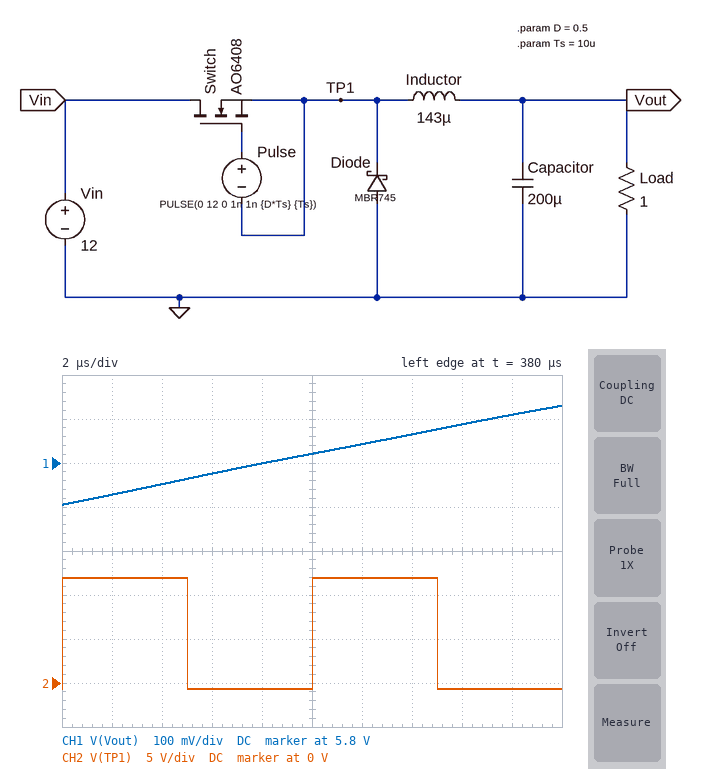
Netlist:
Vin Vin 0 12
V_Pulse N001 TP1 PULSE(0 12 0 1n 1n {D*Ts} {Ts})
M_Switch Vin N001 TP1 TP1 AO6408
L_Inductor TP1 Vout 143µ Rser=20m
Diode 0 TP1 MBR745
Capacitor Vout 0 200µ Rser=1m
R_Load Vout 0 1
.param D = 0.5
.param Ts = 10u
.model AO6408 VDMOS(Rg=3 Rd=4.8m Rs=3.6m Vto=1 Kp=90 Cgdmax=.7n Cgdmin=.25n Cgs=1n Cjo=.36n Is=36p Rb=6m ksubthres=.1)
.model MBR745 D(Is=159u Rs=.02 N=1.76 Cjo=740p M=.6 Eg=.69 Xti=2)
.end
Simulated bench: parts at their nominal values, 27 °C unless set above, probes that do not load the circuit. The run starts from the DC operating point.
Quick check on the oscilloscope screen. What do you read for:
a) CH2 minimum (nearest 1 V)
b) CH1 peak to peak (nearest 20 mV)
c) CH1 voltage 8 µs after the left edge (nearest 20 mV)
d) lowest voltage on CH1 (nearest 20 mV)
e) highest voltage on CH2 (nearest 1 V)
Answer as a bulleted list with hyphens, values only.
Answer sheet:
- -1 V
- 220 mV
- 5.80 V
- 5.70 V
- 12 V
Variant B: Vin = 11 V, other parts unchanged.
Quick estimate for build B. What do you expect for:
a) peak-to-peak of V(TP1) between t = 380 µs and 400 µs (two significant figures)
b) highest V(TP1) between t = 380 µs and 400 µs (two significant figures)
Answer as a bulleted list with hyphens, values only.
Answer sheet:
- 12 V
- 11 V
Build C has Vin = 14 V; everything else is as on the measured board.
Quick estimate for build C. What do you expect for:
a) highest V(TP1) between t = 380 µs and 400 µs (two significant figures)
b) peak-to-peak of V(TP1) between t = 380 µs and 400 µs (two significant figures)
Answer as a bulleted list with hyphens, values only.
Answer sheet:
- 14 V
- 15 V
